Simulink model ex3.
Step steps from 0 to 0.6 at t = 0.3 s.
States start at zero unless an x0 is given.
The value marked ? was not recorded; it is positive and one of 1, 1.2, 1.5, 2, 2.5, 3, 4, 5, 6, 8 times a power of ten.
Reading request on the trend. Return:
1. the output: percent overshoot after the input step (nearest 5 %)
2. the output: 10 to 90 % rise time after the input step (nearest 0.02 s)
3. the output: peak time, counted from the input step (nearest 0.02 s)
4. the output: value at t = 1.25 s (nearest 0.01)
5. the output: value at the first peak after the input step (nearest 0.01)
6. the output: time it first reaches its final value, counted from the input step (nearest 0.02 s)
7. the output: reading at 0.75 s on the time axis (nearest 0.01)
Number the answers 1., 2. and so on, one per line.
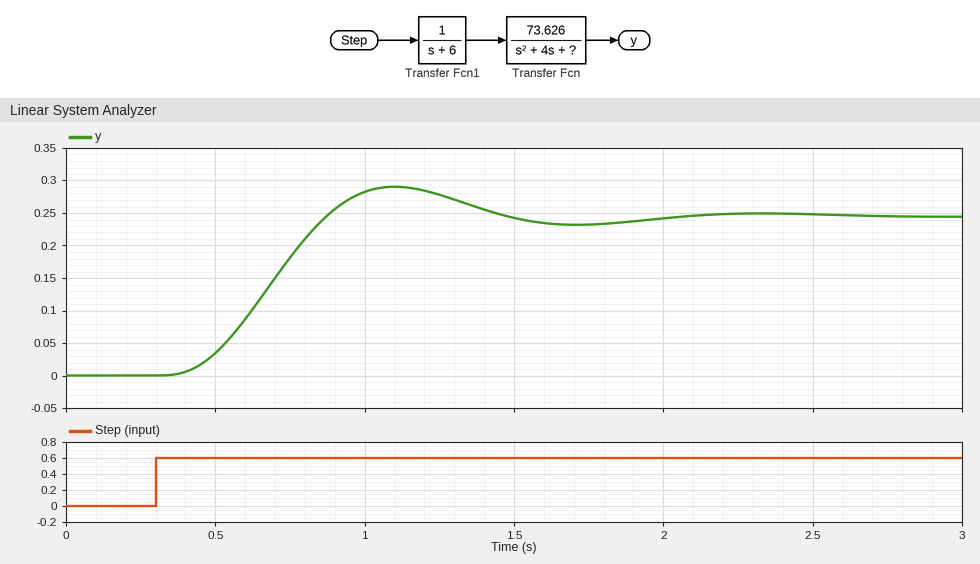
1. 20 %
2. 0.34 s
3. 0.80 s
4. 0.28
5. 0.29
6. 0.58 s
7. 0.18
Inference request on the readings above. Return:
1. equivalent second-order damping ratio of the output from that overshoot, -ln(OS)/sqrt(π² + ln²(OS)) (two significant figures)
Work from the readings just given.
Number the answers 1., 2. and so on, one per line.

1. 0.46
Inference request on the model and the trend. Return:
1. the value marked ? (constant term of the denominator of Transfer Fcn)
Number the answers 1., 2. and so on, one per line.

1. 30
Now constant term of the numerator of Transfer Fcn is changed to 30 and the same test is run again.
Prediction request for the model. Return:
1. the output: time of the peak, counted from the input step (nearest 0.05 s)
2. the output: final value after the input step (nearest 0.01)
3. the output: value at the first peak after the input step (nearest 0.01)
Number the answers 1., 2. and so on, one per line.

1. 0.80 s
2. 0.10
3. 0.12
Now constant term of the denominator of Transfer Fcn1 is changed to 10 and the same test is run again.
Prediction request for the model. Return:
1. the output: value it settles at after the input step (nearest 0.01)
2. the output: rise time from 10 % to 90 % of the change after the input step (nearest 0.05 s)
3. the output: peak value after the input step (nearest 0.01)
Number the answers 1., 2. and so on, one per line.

1. 0.15
2. 0.30 s
3. 0.18
